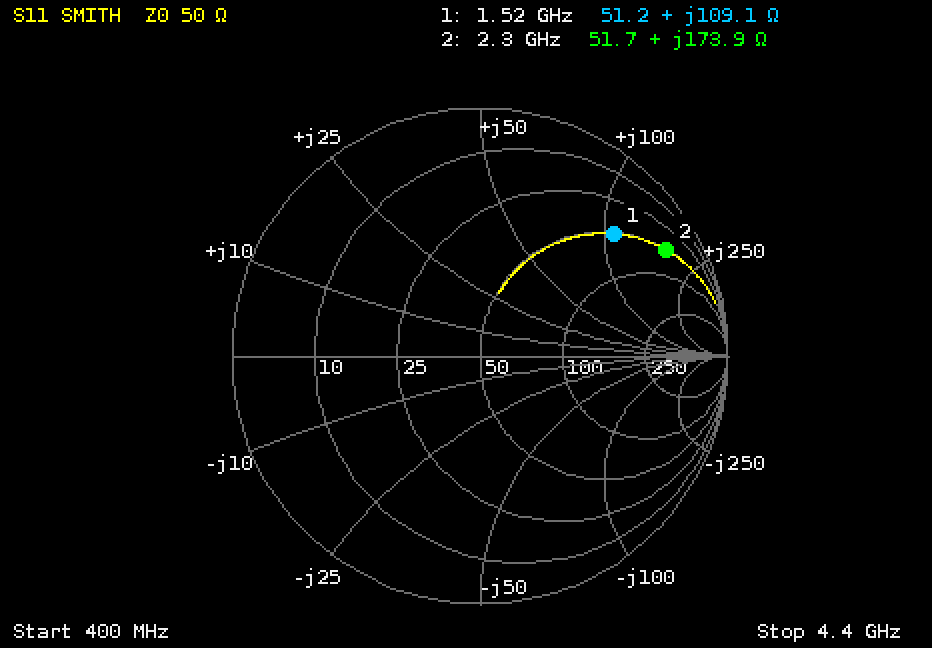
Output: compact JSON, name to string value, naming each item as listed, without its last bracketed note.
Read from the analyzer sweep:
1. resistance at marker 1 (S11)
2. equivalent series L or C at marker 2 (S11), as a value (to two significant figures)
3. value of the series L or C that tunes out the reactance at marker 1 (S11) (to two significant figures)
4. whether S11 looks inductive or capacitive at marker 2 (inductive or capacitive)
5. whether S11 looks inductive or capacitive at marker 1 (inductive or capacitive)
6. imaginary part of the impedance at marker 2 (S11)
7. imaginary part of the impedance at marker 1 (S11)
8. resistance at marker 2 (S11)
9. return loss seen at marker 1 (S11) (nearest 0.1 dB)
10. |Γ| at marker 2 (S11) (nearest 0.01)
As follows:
{"resistance at marker 1": "51.2 Ω", "equivalent series L or C at marker 2 (S11), as a value": "12 nH", "value of the series L or C that tunes out the reactance at marker 1 (S11)": "960 fF", "whether S11 looks inductive or capacitive at marker 2": "inductive", "whether S11 looks inductive or capacitive at marker 1": "inductive", "imaginary part of the impedance at marker 2": "+173.9 Ω", "imaginary part of the impedance at marker 1": "+109.1 Ω", "resistance at marker 2": "51.7 Ω", "return loss seen at marker 1 (S11)": "2.7 dB", "|Γ| at marker 2 (S11)": "0.86"}
